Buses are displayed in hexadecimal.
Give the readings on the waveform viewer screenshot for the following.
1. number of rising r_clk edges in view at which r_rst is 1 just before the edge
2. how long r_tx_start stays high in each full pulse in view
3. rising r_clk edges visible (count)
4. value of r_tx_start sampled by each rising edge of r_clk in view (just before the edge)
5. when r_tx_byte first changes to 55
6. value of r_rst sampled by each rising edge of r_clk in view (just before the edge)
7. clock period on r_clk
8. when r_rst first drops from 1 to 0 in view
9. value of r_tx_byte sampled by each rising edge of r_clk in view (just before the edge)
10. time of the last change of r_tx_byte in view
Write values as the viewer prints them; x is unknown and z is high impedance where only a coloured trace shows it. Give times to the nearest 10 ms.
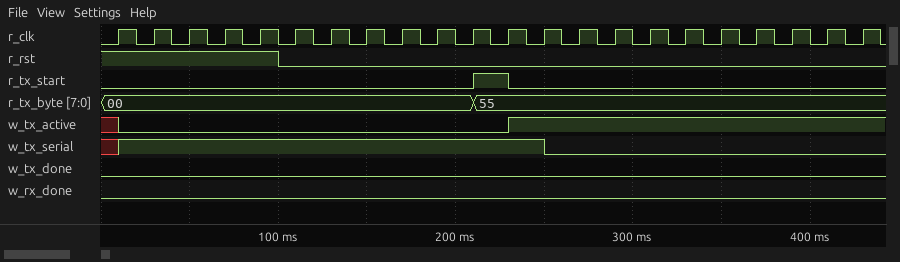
5
20 ms
22
0 0 0 0 0 0 0 0 0 0 0 1 0 0 0 0 0 0 0 0 0 0
210 ms
1 1 1 1 1 0 0 0 0 0 0 0 0 0 0 0 0 0 0 0 0 0
20 ms
100 ms
00, 00, 00, 00, 00, 00, 00, 00, 00, 00, 00, 55, 55, 55, 55, 55, 55, 55, 55, 55, 55, 55
210 ms
